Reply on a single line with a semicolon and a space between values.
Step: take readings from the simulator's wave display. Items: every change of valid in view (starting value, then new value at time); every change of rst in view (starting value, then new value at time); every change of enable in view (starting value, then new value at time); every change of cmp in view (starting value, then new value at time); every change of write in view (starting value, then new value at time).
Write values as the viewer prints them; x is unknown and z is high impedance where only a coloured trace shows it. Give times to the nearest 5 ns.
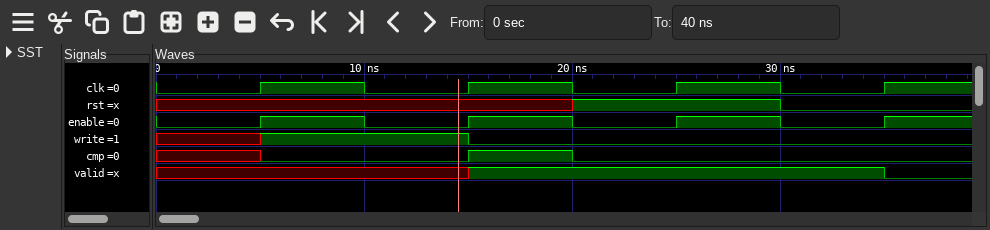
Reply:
x, 1 at 15 ns, 0 at 35 ns; x, 1 at 20 ns, 0 at 30 ns; 0, 1 at 5 ns, 0 at 10 ns, 1 at 15 ns, 0 at 20 ns, 1 at 25 ns, 0 at 30 ns, 1 at 35 ns; x, 0 at 5 ns, 1 at 15 ns, 0 at 20 ns; x, 1 at 5 ns, 0 at 15 ns
